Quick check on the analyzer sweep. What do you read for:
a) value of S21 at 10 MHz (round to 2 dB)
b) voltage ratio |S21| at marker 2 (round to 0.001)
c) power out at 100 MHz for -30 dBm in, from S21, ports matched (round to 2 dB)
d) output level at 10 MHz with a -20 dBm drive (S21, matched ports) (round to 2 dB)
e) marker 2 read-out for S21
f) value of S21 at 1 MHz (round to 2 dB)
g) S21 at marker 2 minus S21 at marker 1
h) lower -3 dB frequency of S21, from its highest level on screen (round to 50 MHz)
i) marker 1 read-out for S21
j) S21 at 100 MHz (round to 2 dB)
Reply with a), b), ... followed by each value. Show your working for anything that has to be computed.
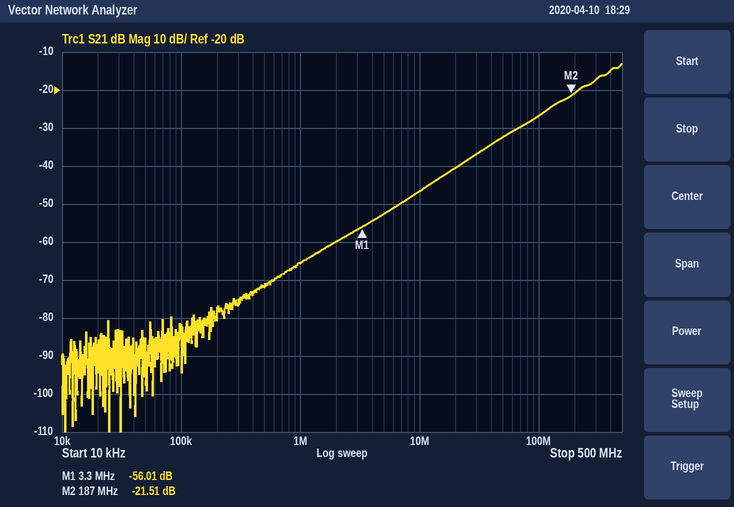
a) -46 dB
b) 10^(-21.51/20) ≈ 0.084
c) -30 dBm + (-26 dB) = -56 dBm
d) -20 dBm + (-46 dB) = -66 dBm
e) -21.51 dB
f) -66 dB
g) -21.51 − (-56.01) = 34.50 dB
h) 350 MHz
i) -56.01 dB
j) -26 dB
